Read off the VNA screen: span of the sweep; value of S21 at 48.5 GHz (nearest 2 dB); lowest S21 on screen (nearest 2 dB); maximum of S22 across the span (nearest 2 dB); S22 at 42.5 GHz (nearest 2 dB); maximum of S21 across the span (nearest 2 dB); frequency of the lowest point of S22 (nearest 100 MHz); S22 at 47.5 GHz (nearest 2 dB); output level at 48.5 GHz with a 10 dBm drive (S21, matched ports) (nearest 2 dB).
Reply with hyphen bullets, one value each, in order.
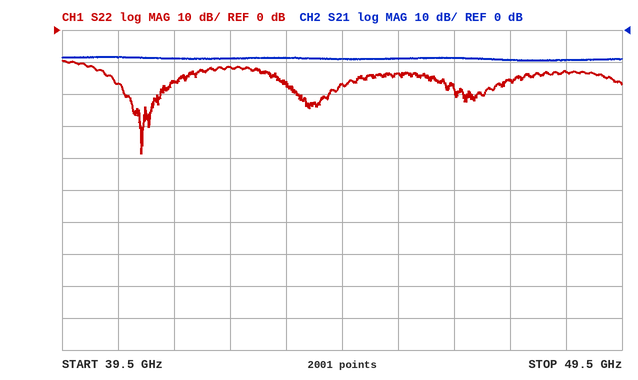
- 10 GHz
- -10 dB
- -10 dB
- -10 dB
- -12 dB
- -8 dB
- 40.9 GHz
- -16 dB
- 0 dBm
